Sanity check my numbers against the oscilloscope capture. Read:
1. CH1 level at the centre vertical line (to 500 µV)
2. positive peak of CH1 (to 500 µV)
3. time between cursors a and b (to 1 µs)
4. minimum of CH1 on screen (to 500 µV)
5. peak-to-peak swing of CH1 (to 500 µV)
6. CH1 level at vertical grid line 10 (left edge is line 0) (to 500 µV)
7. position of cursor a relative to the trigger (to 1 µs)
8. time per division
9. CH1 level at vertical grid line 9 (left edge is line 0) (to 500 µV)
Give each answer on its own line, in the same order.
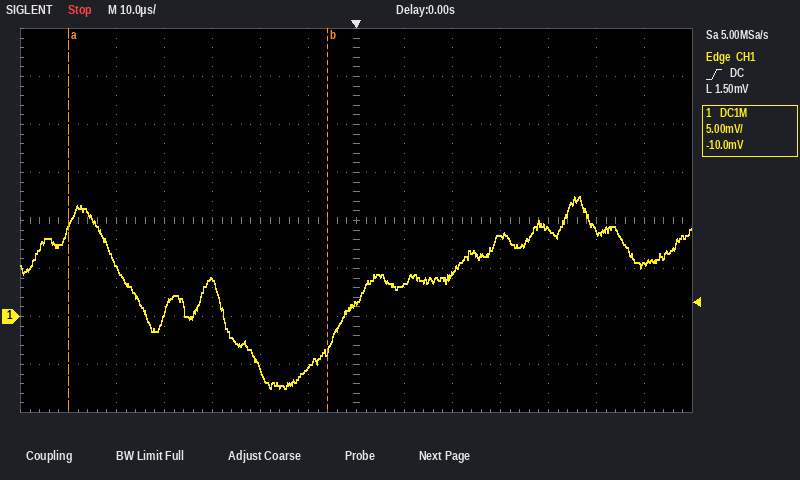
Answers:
1.5 mV
12.5 mV
54 µs
-7.5 mV
20.0 mV
8.5 mV
-60 µs
10 µs
4.5 mV
